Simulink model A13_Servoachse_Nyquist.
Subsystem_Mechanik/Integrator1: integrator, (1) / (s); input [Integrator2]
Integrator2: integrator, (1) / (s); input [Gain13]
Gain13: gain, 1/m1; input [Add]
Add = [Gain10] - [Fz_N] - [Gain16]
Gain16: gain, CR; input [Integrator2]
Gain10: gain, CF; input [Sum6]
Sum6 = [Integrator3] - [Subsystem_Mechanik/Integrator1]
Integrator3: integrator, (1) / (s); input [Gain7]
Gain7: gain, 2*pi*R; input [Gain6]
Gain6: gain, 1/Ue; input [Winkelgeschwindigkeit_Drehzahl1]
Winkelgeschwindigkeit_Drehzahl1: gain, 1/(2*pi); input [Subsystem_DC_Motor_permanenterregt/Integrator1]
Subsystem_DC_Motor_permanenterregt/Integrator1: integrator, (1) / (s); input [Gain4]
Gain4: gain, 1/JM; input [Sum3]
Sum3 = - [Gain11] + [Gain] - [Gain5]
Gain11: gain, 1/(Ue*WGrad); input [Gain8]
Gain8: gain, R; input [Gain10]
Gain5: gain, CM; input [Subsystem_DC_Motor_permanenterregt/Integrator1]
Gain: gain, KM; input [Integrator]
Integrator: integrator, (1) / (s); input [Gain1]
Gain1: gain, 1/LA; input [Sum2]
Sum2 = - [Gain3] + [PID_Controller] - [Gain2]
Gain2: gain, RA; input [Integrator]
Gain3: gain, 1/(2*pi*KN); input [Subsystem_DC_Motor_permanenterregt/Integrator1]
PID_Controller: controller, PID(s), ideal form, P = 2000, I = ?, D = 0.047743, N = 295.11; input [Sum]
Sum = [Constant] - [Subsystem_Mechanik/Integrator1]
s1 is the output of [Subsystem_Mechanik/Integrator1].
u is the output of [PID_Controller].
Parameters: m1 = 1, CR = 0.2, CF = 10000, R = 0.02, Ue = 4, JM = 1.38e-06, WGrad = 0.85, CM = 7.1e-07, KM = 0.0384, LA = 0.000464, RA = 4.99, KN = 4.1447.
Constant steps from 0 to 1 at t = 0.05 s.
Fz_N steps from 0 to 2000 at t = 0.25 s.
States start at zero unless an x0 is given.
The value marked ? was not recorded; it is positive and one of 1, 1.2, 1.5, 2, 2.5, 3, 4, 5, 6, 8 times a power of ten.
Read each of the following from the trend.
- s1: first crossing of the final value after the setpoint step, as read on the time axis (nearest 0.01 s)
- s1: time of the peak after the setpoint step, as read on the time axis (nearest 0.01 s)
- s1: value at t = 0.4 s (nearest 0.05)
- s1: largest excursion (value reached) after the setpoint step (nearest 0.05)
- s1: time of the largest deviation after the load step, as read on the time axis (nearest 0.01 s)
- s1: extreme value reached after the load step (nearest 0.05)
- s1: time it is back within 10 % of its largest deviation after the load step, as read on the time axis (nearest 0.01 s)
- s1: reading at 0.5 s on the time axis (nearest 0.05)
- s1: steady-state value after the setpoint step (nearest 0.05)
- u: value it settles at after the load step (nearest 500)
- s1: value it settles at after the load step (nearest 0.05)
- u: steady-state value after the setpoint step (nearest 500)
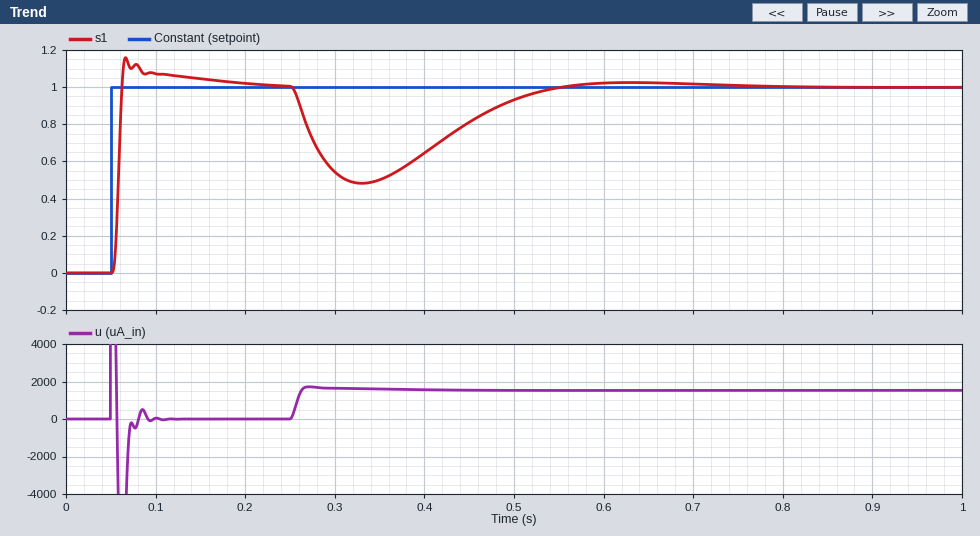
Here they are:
0.06 s
0.07 s
0.65
1.15
0.33 s
0.50
0.51 s
0.95
1.00
1500
1.00
0
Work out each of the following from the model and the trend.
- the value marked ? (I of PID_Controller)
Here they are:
10
